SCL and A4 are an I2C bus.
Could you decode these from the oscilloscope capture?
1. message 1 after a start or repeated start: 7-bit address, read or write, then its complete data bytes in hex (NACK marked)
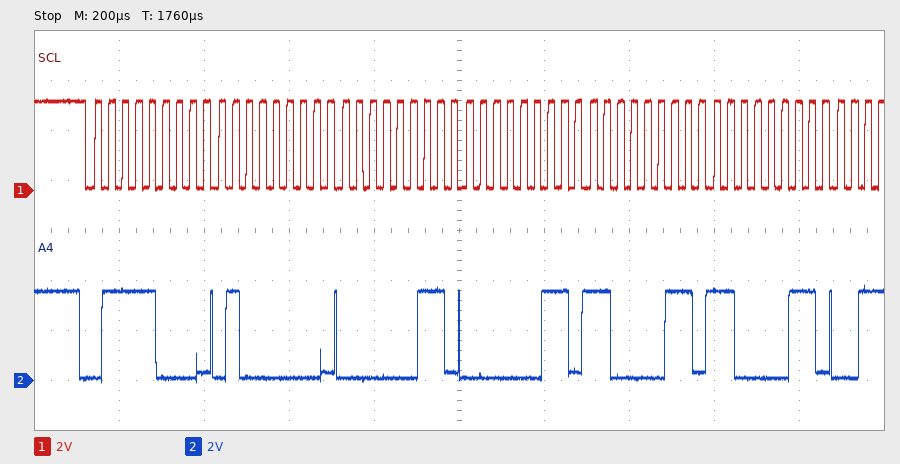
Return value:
0x3C write: 40 03 03 C3 C3
